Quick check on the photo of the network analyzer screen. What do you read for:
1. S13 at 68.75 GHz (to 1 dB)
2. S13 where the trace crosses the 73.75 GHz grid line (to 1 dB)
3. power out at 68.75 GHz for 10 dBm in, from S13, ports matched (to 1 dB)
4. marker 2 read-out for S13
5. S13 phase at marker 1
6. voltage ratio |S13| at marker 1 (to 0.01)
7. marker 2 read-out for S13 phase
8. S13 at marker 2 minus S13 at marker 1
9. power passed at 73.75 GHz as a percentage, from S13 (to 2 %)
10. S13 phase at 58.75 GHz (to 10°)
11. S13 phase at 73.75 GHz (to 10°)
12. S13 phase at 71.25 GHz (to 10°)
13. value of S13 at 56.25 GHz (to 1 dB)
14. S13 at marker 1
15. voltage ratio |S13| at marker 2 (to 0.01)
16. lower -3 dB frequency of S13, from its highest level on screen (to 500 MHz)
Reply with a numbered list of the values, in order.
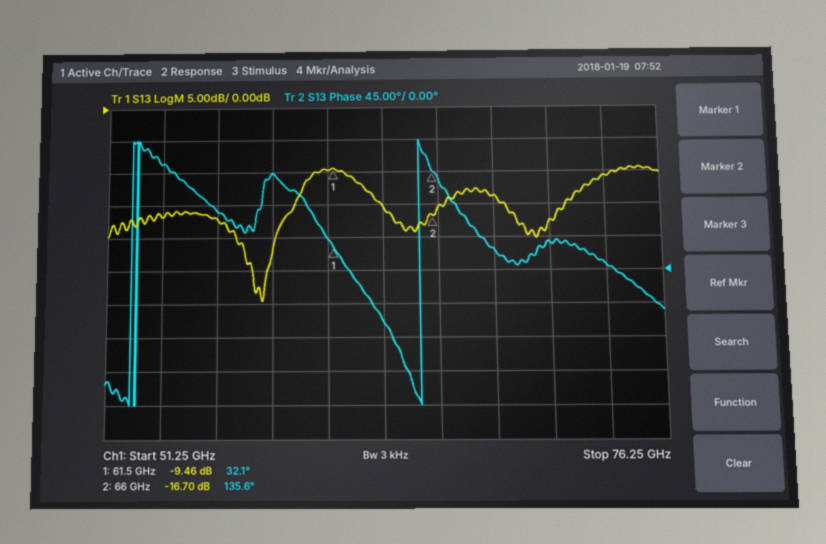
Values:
1. -14 dB
2. -11 dB
3. -4 dBm
4. -16.70 dB
5. 32.1°
6. 0.34
7. 135.6°
8. -7.24 dB
9. 8 %
10. 130°
11. 10°
12. 40°
13. -17 dB
14. -9.46 dB
15. 0.15
16. 60.0 GHz
